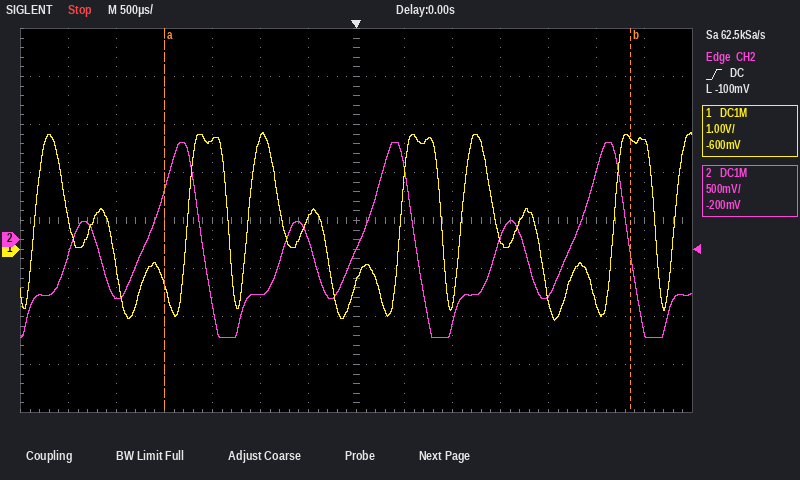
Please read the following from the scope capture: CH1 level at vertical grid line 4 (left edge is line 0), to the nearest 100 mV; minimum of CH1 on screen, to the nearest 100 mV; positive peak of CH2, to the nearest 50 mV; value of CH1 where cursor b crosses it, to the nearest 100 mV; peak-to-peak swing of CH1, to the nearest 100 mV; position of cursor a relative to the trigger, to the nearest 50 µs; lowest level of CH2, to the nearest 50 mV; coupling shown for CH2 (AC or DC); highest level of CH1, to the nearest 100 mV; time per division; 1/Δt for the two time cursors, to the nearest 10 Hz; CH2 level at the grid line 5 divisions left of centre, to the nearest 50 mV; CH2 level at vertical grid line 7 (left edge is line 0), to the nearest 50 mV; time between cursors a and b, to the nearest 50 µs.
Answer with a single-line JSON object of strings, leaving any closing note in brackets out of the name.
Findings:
{"CH1 level at vertical grid line 4 (left edge is line 0), to the nearest 100 mV": "2.3 V", "minimum of CH1 on screen, to the nearest 100 mV": "-1.5 V", "positive peak of CH2, to the nearest 50 mV": "1.00 V", "value of CH1 where cursor b crosses it, to the nearest 100 mV": "2.3 V", "peak-to-peak swing of CH1, to the nearest 100 mV": "3.9 V", "position of cursor a relative to the trigger, to the nearest 50 µs": "-2.00 ms", "lowest level of CH2, to the nearest 50 mV": "-1.00 V", "coupling shown for CH2": "DC", "highest level of CH1, to the nearest 100 mV": "2.4 V", "time per division": "500 µs", "1/Δt for the two time cursors, to the nearest 10 Hz": "210 Hz", "CH2 level at the grid line 5 divisions left of centre, to the nearest 50 mV": "-600 mV", "CH2 level at vertical grid line 7 (left edge is line 0), to the nearest 50 mV": "-100 mV", "time between cursors a and b, to the nearest 50 µs": "4.85 ms"}
